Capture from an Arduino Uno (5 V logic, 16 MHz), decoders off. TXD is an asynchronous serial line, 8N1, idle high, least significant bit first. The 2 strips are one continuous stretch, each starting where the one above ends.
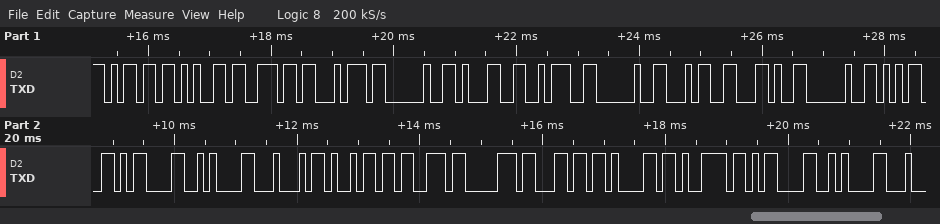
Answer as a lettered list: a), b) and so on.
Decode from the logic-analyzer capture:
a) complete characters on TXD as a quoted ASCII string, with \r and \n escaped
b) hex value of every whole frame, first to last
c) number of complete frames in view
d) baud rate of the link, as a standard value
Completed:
a) "ment 1: 4, 5\r\nDisplay\r\n"
b) 6D 65 6E 74 20 31 3A 20 34 2C 20 35 0D 0A 44 69 73 70 6C 61 79 0D 0A
c) 23
d) 9600 baud
